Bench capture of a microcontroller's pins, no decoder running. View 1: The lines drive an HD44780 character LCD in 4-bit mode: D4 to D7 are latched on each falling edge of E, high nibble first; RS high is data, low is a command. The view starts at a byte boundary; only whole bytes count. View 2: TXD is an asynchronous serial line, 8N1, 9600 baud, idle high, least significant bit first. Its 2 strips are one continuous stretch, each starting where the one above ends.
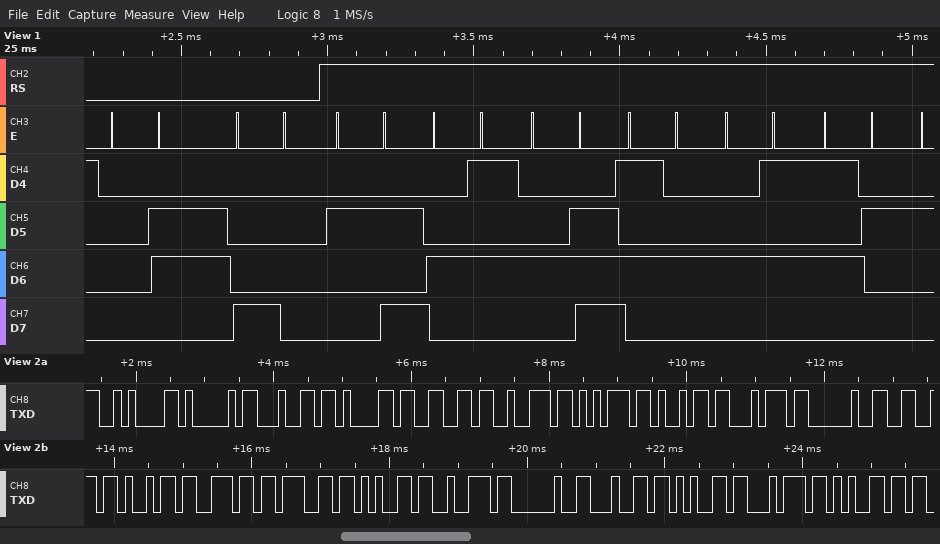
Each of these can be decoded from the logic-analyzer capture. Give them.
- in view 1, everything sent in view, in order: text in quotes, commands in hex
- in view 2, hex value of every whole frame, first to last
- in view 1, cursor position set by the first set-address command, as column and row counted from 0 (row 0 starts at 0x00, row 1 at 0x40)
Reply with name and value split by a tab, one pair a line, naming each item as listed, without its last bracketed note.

in view 1, everything sent in view, in order: text in quotes, commands in hex	0x06 0x80 "*ENTER"
in view 2, hex value of every whole frame, first to last	0A 41 64 61 66 72 75 69 74 20 66 69 6E 67 65 72 20 64 65 74 65
in view 1, cursor position set by the first set-address command, as column and row counted from 0	column 0, row 0
